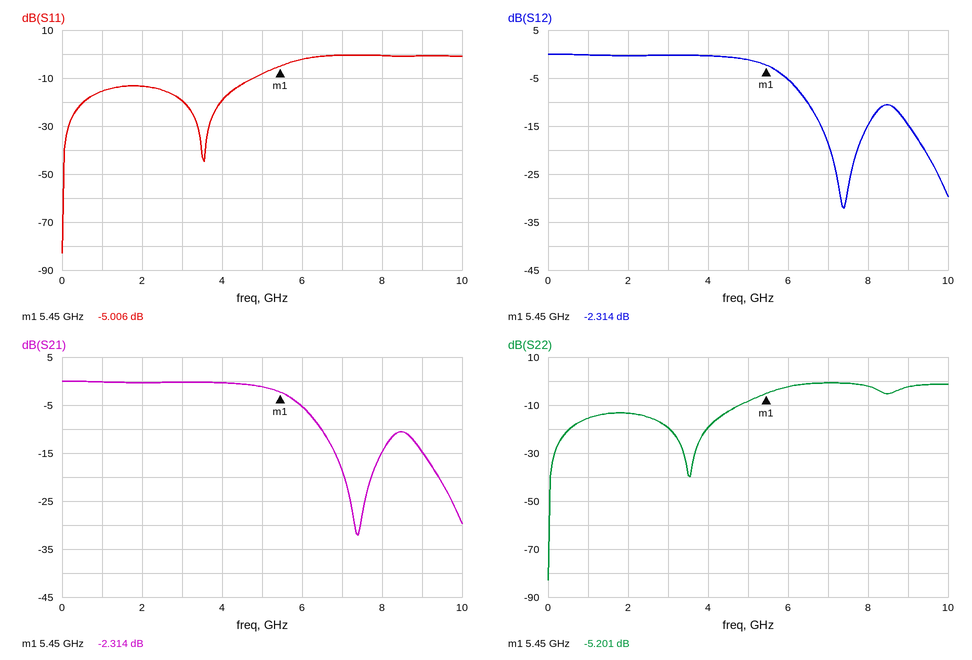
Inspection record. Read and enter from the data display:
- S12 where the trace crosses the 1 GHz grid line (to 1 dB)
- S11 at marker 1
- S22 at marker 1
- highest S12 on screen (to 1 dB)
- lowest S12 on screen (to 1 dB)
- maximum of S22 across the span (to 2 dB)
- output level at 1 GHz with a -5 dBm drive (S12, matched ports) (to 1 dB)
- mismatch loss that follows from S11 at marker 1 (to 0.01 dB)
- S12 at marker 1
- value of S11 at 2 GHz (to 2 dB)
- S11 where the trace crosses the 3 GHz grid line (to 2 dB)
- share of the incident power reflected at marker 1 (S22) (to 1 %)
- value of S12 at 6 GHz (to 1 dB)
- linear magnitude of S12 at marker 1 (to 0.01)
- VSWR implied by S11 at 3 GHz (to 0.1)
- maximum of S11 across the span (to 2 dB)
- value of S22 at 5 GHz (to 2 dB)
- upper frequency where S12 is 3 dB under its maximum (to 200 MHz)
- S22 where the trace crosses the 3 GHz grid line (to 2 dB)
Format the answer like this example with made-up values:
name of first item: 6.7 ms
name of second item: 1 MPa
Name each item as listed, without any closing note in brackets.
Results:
S12 where the trace crosses the 1 GHz grid line: 0 dB
S11 at marker 1: -5.006 dB
S22 at marker 1: -5.201 dB
highest S12 on screen: 0 dB
lowest S12 on screen: -32 dB
maximum of S22 across the span: 0 dB
output level at 1 GHz with a -5 dBm drive (S12, matched ports): -5 dBm
mismatch loss that follows from S11 at marker 1: 1.65 dB
S12 at marker 1: -2.314 dB
value of S11 at 2 GHz: -14 dB
S11 where the trace crosses the 3 GHz grid line: -20 dB
share of the incident power reflected at marker 1 (S22): 30 %
value of S12 at 6 GHz: -5 dB
linear magnitude of S12 at marker 1: 0.77
VSWR implied by S11 at 3 GHz: 1.2
maximum of S11 across the span: 0 dB
value of S22 at 5 GHz: -8 dB
upper frequency where S12 is 3 dB under its maximum: 5.6 GHz
S22 where the trace crosses the 3 GHz grid line: -20 dB
